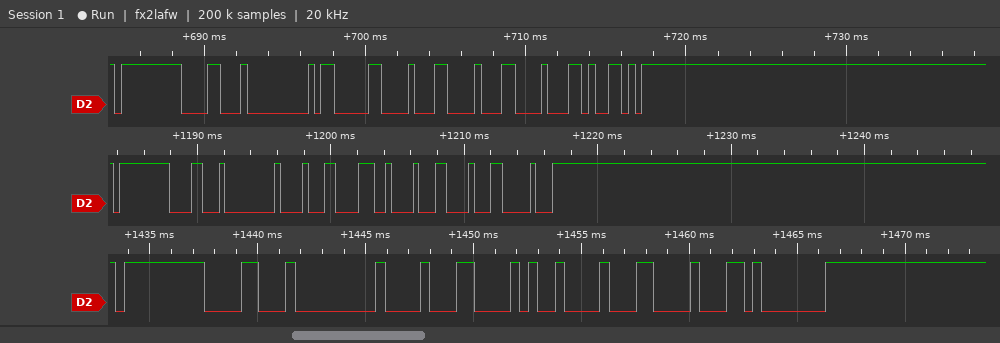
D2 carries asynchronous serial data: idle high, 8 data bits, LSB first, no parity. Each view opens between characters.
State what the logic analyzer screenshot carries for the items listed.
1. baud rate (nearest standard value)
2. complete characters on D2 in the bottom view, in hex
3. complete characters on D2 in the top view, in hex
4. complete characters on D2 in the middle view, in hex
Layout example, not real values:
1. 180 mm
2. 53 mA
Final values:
1. 2400 baud
2. FF, 18, 00, 88, 28, 88, 88, 01
3. FF, 18, 00, 83, 88, 88, 88, 59
4. FF, 18, 00, 88, 38, 88, 88, 10
